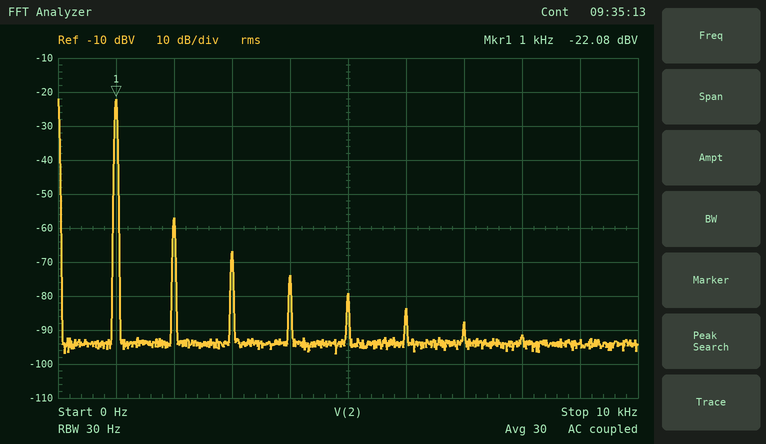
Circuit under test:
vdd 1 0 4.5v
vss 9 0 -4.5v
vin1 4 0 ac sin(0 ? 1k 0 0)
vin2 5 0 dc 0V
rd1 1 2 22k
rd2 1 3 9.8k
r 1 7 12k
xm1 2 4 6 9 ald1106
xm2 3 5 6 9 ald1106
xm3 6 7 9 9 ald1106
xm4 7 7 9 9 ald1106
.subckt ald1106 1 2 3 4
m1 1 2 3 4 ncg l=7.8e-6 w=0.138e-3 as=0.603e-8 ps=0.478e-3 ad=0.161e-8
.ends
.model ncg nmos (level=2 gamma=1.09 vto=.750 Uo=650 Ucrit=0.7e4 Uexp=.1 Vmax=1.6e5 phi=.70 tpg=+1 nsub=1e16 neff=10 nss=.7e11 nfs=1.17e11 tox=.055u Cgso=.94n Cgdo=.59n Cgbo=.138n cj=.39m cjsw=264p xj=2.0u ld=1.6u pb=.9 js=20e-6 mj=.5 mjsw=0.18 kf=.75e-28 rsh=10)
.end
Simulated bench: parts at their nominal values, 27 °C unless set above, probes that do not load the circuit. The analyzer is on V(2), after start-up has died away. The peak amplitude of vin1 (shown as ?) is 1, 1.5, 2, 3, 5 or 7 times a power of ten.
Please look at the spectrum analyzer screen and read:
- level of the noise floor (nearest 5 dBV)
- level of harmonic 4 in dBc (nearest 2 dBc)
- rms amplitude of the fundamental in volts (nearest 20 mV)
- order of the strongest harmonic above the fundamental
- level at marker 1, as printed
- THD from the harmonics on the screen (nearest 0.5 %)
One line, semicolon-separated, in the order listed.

-95 dBV; -52 dBc; 80 mV; 2; -22.08 dBV; 2.0 %
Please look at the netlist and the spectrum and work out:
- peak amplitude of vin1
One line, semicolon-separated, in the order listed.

20 mV
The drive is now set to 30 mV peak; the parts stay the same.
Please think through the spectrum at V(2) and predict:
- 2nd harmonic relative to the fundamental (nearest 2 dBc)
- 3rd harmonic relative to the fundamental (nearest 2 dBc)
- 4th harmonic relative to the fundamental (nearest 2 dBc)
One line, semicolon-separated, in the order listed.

-26 dBc; -32 dBc; -42 dBc
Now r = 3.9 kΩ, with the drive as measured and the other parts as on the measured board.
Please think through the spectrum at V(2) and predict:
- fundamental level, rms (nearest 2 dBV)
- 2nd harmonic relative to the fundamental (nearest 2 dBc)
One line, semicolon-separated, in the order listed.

-62 dBV; -48 dBc
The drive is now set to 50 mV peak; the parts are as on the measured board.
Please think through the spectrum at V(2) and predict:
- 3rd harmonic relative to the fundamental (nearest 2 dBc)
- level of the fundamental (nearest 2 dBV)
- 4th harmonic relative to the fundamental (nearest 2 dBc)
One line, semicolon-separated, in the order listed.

-28 dBc; -16 dBV; -50 dBc
